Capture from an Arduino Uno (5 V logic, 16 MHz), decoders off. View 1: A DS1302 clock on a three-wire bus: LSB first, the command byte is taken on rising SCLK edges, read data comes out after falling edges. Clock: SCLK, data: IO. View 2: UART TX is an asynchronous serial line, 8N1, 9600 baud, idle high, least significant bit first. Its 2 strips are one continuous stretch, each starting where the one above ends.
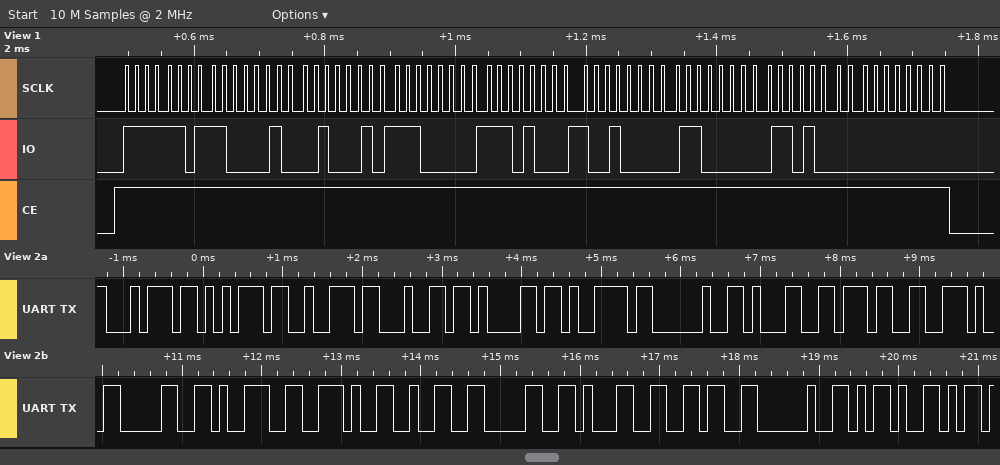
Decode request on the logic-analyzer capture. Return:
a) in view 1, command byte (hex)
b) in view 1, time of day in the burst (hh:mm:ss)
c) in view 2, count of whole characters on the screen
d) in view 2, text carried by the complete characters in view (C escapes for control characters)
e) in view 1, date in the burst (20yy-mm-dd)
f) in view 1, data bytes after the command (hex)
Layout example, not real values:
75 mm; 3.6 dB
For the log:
0xBF; 07:44:43; 19; "turday 17.09.2016 -"; 2016-09-17; 43 44 07 17 09 06 16 00
